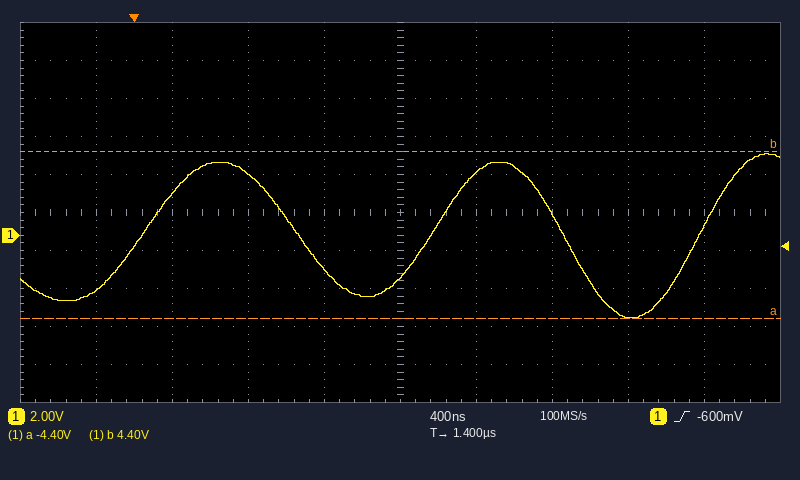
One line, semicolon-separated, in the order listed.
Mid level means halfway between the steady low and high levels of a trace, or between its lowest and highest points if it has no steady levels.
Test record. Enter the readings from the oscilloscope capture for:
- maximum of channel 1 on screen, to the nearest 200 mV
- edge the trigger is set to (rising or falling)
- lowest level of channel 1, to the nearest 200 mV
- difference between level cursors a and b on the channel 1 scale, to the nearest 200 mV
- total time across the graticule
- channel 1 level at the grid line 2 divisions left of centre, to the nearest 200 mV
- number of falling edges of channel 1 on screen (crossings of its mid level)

4.4 V; rising; -4.4 V; 8.8 V; 4 µs; 3.2 V; 2
